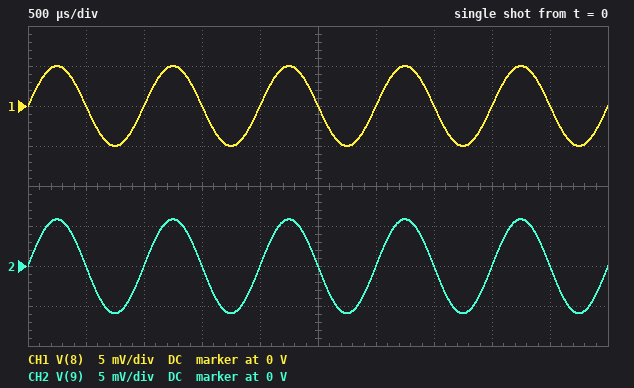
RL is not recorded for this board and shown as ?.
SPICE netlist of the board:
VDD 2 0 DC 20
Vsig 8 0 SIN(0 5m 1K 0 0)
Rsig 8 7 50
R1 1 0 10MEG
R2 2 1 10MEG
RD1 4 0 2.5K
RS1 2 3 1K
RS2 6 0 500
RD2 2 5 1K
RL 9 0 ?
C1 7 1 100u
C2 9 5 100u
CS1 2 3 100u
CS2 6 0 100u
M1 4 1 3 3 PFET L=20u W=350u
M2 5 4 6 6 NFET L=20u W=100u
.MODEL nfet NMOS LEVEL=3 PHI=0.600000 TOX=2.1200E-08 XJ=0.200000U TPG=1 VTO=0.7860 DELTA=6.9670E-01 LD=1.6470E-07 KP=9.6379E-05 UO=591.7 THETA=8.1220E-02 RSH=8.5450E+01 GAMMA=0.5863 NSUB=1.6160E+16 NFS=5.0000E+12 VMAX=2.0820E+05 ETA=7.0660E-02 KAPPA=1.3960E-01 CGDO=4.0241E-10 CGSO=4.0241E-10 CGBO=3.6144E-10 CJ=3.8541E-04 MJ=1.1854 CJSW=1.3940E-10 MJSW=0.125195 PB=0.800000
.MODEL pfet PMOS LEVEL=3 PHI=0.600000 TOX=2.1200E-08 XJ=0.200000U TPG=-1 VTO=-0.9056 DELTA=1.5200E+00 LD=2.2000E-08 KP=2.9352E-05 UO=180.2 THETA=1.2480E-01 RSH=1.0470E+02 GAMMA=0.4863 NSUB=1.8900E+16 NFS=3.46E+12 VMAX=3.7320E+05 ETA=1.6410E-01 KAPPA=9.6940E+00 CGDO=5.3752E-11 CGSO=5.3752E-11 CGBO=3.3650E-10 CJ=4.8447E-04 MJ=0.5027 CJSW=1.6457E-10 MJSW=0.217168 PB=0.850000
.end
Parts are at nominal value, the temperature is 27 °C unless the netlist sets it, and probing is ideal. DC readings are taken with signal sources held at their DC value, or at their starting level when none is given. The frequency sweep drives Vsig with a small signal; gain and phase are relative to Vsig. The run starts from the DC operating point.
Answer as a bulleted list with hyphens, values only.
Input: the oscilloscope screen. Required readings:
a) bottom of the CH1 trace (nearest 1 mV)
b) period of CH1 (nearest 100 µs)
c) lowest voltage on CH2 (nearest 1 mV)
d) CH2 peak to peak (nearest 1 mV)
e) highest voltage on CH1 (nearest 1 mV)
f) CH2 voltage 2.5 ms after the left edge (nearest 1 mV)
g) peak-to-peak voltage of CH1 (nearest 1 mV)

- -5 mV
- 1.0 ms
- -6 mV
- 12 mV
- 5 mV
- 0 V
- 10 mV
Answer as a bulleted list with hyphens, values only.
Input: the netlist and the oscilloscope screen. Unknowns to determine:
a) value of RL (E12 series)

- 680 Ω
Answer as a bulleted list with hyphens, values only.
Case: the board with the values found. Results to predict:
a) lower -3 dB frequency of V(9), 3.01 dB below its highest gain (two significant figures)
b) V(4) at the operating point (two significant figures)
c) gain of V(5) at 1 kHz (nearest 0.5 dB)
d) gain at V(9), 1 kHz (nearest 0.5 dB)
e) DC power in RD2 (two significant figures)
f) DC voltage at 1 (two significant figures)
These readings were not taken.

- 4.7 Hz
- 8.9 V
- 1.5 dB
- 1.5 dB
- 18 mW
- 10 V
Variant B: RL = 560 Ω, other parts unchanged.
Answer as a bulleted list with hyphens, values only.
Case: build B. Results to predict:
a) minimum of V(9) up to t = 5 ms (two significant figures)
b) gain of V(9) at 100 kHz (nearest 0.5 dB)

- -5.2 mV
- 0.5 dB
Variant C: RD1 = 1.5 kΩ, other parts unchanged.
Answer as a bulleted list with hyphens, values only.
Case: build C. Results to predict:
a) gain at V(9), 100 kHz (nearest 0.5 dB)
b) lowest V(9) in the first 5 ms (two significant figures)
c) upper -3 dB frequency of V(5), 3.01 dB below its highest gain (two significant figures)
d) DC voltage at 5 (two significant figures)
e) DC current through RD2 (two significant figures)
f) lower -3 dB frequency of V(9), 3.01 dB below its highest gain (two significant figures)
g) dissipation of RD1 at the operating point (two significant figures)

- -5.5 dB
- -2.7 mV
- 44 MHz
- 18 V
- 1.9 mA
- 4.2 Hz
- 19 mW
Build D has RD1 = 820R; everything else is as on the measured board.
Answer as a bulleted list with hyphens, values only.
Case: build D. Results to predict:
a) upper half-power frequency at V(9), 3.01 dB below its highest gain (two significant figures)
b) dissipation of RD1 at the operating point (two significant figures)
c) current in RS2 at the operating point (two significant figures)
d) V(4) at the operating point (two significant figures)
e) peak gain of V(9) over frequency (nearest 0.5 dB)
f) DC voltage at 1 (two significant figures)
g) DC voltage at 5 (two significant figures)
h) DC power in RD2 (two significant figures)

- 68 MHz
- 10 mW
- 570 µA
- 2.9 V
- -14.5 dB
- 10 V
- 19 V
- 330 µW
